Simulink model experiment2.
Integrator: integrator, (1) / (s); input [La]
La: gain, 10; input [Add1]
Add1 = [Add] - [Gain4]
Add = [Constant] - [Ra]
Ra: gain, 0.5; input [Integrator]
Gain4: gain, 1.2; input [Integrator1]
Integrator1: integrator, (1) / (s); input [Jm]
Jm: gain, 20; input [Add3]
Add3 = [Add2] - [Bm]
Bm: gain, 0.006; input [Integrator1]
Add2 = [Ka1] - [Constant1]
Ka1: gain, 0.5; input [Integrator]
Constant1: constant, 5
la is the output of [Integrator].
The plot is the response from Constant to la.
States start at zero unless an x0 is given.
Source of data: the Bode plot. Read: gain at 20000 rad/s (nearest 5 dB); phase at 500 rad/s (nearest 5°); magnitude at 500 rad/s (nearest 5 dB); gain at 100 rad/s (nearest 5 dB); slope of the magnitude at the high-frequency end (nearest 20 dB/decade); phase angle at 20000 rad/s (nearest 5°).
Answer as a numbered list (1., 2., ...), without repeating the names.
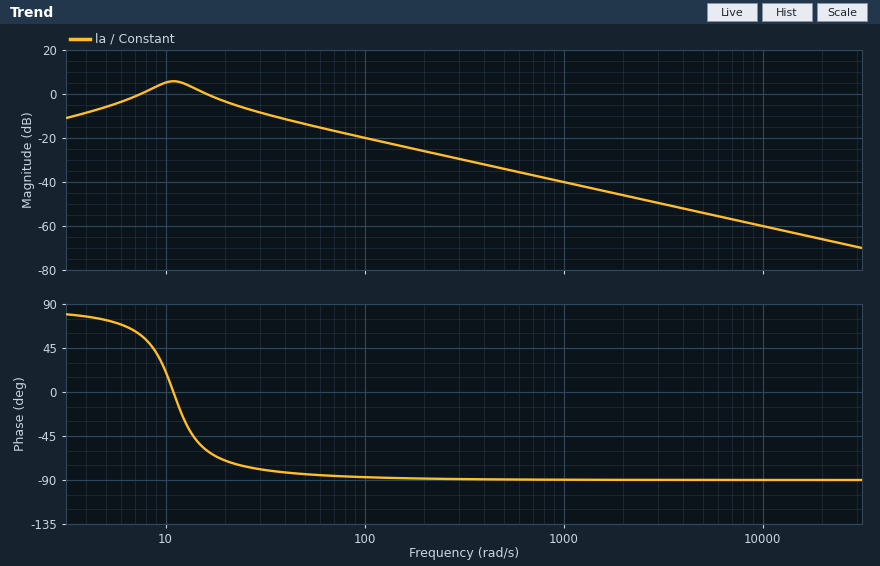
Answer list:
1. -65 dB
2. -90°
3. -35 dB
4. -20 dB
5. -20 dB/decade
6. -90°
